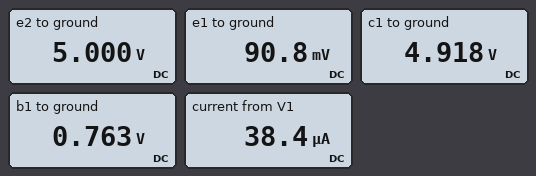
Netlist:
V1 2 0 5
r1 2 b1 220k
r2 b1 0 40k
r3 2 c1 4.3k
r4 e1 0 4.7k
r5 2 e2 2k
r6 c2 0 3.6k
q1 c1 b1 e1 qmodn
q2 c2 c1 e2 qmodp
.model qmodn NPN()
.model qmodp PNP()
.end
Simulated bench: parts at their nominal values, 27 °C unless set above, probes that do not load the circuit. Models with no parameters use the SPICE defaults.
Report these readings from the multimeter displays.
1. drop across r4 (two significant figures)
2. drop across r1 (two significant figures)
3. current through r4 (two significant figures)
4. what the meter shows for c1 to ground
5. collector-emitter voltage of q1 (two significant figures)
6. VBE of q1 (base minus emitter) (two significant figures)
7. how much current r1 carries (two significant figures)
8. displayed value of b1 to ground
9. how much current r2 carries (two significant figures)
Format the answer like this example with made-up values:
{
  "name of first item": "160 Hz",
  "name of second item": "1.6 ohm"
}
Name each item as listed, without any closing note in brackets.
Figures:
{
  "drop across r4": "91 mV",
  "drop across r1": "4.2 V",
  "current through r4": "19 µA",
  "what the meter shows for c1 to ground": "4.918 V",
  "collector-emitter voltage of q1": "4.8 V",
  "VBE of q1 (base minus emitter)": "670 mV",
  "how much current r1 carries": "19 µA",
  "displayed value of b1 to ground": "0.763 V",
  "how much current r2 carries": "19 µA"
}
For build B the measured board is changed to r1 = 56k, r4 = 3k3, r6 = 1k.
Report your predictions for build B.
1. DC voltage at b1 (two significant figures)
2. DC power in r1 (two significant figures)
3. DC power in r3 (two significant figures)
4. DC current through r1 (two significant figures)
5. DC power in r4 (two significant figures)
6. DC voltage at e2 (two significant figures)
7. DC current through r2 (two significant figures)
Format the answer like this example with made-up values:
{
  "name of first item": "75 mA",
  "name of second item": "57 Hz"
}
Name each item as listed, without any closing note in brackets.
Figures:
{
  "DC voltage at b1": "2.0 V",
  "DC power in r1": "160 µW",
  "DC power in r3": "590 µW",
  "DC current through r1": "54 µA",
  "DC power in r4": "470 µW",
  "DC voltage at e2": "4.2 V",
  "DC current through r2": "50 µA"
}
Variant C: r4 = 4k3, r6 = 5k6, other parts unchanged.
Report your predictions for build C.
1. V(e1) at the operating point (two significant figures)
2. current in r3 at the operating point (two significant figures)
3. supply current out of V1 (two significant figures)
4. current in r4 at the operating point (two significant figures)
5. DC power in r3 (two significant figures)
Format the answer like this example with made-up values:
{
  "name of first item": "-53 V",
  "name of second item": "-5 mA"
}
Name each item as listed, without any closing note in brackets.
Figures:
{
  "V(e1) at the operating point": "89 mV",
  "current in r3 at the operating point": "20 µA",
  "supply current out of V1": "40 µA",
  "current in r4 at the operating point": "21 µA",
  "DC power in r3": "1.8 µW"
}
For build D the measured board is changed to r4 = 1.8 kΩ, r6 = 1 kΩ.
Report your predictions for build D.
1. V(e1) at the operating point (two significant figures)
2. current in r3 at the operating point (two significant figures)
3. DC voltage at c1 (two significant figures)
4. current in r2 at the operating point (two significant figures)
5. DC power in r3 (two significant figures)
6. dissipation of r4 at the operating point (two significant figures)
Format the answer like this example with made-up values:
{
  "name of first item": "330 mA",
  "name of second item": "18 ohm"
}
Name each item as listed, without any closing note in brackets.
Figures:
{
  "V(e1) at the operating point": "68 mV",
  "current in r3 at the operating point": "37 µA",
  "DC voltage at c1": "4.8 V",
  "current in r2 at the operating point": "19 µA",
  "DC power in r3": "5.9 µW",
  "dissipation of r4 at the operating point": "2.5 µW"
}
